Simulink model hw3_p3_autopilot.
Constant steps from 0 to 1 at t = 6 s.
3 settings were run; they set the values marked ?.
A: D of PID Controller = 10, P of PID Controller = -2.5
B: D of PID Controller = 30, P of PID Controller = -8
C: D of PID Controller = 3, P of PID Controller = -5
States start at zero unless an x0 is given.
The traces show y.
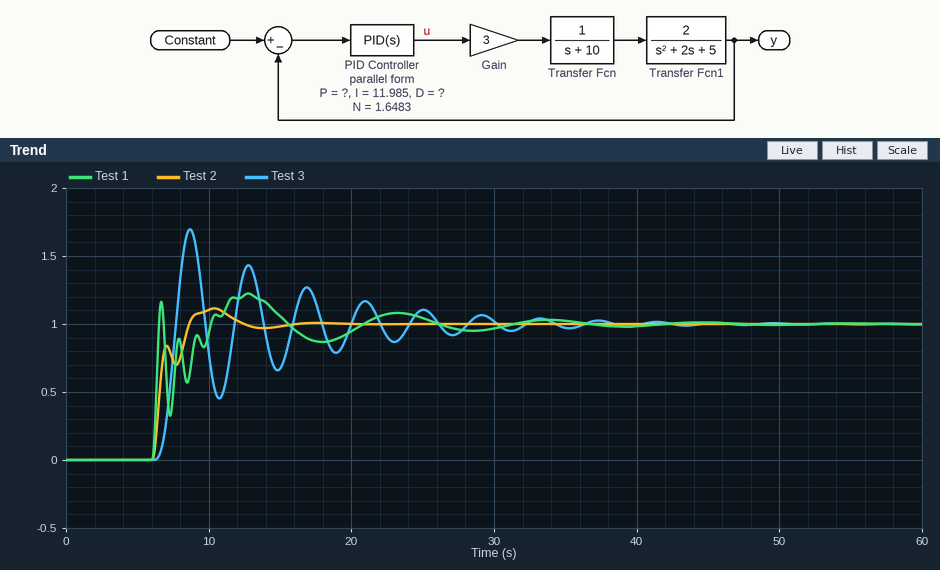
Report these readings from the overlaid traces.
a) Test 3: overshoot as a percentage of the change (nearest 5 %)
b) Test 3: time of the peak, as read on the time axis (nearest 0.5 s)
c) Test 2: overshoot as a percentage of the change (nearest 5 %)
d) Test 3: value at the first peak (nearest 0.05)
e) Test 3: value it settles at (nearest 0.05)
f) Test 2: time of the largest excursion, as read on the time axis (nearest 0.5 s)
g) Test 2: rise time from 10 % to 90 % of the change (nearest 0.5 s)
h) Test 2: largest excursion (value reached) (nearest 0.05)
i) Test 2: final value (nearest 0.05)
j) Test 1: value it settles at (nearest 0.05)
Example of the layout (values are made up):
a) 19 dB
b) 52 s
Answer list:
a) 70 %
b) 8.5 s
c) 10 %
d) 1.70
e) 1.00
f) 10.5 s
g) 2.0 s
h) 1.10
i) 1.00
j) 1.00
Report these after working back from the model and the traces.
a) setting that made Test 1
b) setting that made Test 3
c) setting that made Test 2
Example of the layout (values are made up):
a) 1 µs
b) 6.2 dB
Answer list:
a) B
b) C
c) A
